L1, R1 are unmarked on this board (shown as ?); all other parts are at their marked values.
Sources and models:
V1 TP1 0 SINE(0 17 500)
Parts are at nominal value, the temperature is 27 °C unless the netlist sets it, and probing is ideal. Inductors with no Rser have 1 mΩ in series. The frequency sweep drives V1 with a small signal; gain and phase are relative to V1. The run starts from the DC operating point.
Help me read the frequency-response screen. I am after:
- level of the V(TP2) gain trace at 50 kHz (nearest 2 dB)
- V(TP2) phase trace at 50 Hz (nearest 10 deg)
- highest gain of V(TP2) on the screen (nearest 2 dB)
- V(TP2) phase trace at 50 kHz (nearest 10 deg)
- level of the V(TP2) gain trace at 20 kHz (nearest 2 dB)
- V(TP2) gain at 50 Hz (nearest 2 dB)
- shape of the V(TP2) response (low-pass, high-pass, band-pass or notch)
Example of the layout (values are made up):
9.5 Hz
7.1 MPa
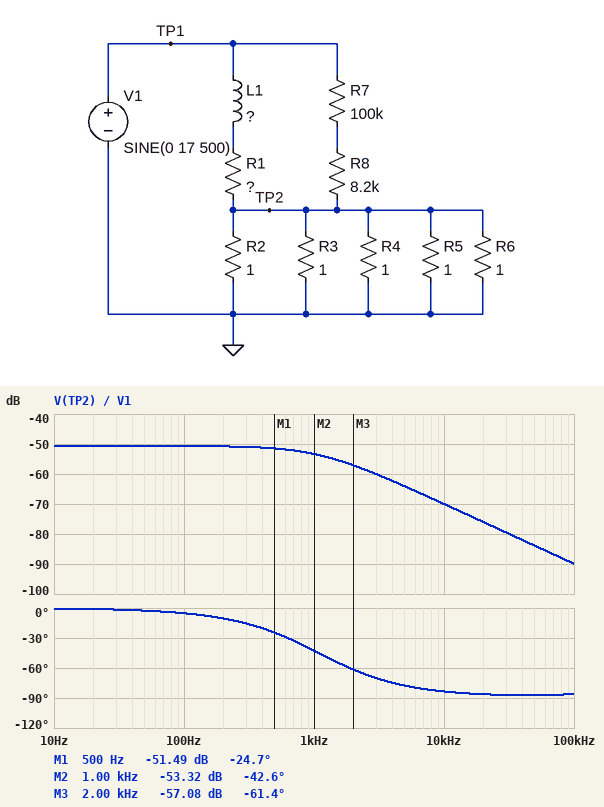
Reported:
-84 dB
0 deg
-50 dB
-90 deg
-76 dB
-50 dB
low-pass
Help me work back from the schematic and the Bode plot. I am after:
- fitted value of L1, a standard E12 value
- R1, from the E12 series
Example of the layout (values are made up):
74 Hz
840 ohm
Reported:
10 mH
68 Ω
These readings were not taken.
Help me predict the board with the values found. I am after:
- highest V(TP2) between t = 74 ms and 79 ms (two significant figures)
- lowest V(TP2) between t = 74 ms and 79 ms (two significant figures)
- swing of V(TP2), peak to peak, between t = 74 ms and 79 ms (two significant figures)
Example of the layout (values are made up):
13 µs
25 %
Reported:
45 mV
-45 mV
91 mV
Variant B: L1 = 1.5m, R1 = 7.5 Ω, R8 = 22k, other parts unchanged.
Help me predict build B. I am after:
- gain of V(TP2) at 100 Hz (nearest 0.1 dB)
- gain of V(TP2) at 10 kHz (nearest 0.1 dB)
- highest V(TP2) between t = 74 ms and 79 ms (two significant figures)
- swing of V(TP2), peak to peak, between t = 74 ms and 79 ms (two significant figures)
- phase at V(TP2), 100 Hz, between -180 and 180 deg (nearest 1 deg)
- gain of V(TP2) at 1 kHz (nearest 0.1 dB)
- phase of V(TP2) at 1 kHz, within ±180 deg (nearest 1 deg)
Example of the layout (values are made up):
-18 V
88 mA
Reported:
-31.8 dB
-53.5 dB
380 mV
750 mV
-7 deg
-35.7 dB
-51 deg
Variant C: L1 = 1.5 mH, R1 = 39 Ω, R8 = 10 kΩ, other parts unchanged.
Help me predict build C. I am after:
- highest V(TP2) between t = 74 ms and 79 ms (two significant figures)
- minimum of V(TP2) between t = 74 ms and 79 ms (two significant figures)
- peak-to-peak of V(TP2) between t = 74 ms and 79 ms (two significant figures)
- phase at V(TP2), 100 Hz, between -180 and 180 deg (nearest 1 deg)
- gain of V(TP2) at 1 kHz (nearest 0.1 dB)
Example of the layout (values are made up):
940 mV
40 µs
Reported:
86 mV
-86 mV
170 mV
-1 deg
-46.1 dB
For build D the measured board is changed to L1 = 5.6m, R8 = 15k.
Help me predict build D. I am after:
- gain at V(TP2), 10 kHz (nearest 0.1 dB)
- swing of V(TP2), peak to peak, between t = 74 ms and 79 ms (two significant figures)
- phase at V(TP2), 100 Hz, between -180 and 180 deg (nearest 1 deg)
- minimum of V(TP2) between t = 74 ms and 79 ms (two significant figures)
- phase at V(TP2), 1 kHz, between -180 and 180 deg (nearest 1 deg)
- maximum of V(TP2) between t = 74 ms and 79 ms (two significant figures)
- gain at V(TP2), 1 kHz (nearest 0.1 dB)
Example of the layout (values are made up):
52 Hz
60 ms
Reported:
-65.1 dB
97 mV
-3 deg
-48 mV
-27 deg
48 mV
-51.7 dB
